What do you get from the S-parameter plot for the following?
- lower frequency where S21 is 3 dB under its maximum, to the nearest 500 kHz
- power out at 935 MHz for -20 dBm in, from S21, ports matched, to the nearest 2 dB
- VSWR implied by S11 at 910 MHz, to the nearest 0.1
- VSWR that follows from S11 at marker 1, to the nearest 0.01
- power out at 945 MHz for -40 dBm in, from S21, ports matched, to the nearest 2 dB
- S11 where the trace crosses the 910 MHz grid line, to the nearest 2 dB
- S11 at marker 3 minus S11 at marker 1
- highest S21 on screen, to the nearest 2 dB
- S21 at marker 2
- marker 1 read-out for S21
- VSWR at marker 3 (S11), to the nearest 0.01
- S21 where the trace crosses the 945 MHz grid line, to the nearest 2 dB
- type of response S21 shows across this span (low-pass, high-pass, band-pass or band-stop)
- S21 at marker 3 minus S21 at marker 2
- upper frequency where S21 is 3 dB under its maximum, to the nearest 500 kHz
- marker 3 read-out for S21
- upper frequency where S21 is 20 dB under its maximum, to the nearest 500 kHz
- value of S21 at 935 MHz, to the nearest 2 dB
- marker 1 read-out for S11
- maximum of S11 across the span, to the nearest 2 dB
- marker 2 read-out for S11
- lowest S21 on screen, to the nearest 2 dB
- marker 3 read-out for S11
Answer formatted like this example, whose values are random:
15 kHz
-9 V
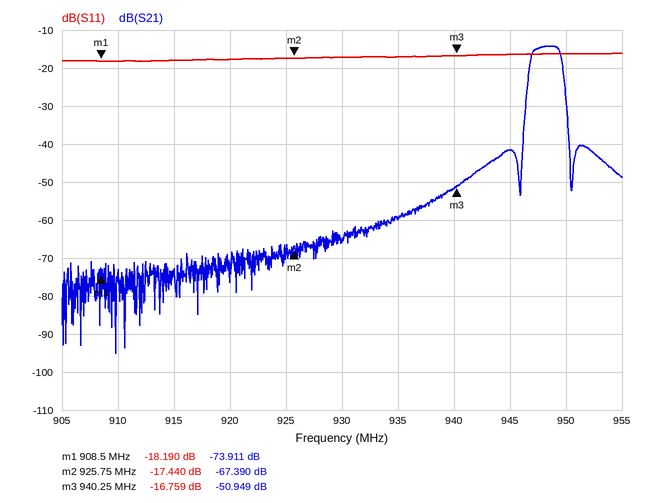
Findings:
947.0 MHz
-80 dBm
1.3
1.28
-82 dBm
-18 dB
1.431 dB
-14 dB
-67.390 dB
-73.911 dB
1.34
-42 dB
band-pass
16.441 dB
949.5 MHz
-50.949 dB
950.0 MHz
-60 dB
-18.190 dB
-16 dB
-17.440 dB
-96 dB
-16.759 dB
